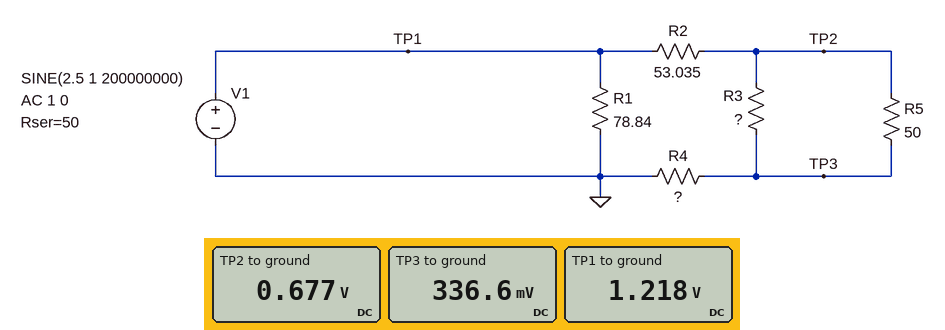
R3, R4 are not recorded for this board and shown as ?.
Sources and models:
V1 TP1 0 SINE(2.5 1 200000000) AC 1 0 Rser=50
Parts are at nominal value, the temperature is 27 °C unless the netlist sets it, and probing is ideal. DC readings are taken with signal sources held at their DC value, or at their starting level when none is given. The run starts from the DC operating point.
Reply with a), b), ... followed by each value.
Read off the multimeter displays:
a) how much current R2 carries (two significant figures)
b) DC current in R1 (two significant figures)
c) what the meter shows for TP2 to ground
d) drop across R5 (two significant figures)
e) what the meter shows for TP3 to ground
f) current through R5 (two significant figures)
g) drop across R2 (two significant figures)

a) 10 mA
b) 15 mA
c) 0.677 V
d) 340 mV
e) 336.6 mV
f) 6.8 mA
g) 540 mV
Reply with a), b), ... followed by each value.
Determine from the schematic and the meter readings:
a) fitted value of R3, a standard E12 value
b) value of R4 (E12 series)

a) 100 Ω
b) 33 Ω
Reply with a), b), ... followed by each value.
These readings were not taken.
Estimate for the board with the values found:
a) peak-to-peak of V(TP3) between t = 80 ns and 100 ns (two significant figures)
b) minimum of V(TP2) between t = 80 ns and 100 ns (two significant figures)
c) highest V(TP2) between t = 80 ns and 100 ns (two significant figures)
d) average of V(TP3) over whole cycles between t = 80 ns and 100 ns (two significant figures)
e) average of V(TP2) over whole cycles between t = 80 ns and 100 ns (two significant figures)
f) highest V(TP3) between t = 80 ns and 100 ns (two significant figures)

a) 270 mV
b) 410 mV
c) 950 mV
d) 340 mV
e) 680 mV
f) 470 mV
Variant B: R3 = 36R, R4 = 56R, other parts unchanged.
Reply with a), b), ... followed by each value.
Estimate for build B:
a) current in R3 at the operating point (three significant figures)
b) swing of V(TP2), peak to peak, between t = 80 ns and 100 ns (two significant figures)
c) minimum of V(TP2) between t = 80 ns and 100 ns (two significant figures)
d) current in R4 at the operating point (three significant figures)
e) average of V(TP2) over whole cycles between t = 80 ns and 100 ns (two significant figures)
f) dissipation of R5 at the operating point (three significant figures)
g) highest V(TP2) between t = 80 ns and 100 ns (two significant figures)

a) 5.54 mA
b) 590 mV
c) 440 mV
d) 9.53 mA
e) 730 mV
f) 795 µW
g) 1.0 V
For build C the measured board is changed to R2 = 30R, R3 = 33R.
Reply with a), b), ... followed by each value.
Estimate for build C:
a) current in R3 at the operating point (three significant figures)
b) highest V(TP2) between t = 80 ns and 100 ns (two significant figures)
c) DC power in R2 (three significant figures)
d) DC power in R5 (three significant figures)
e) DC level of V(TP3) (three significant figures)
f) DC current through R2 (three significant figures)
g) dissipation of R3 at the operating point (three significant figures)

a) 8.12 mA
b) 1.0 V
c) 5.45 mW
d) 1.44 mW
e) 445 mV
f) 13.5 mA
g) 2.18 mW
